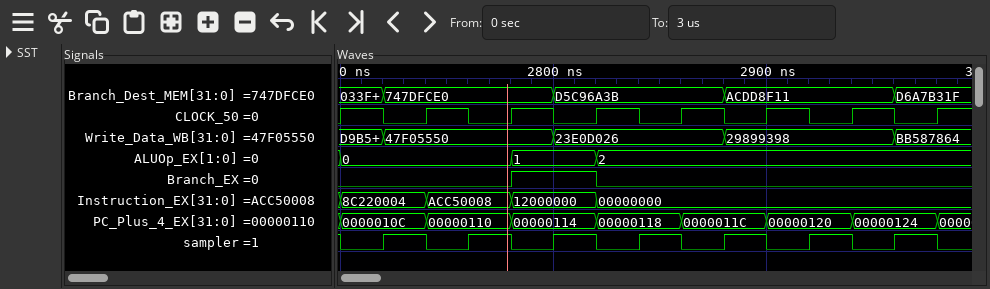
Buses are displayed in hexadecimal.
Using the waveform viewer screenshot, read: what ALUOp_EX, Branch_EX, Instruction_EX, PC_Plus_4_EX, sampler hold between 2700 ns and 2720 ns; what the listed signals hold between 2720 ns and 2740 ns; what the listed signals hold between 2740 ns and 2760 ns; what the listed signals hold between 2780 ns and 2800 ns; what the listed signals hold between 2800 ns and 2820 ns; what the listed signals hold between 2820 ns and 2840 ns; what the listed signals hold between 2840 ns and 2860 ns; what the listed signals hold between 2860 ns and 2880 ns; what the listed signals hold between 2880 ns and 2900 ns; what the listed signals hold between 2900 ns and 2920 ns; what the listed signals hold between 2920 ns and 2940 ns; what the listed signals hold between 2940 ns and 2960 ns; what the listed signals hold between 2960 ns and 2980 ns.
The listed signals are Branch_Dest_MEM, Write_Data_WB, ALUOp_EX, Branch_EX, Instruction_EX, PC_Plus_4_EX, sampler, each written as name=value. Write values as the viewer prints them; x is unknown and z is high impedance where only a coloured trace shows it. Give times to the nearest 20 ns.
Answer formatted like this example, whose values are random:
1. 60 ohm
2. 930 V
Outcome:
1. ALUOp_EX=0, Branch_EX=0, Instruction_EX=8C220004, PC_Plus_4_EX=0000010C, sampler=0
2. Branch_Dest_MEM=747DFCE0, Write_Data_WB=47F05550, ALUOp_EX=0, Branch_EX=0, Instruction_EX=8C220004, PC_Plus_4_EX=0000010C, sampler=1
3. Branch_Dest_MEM=747DFCE0, Write_Data_WB=47F05550, ALUOp_EX=0, Branch_EX=0, Instruction_EX=ACC50008, PC_Plus_4_EX=00000110, sampler=0
4. Branch_Dest_MEM=747DFCE0, Write_Data_WB=47F05550, ALUOp_EX=1, Branch_EX=1, Instruction_EX=12000000, PC_Plus_4_EX=00000114, sampler=0
5. Branch_Dest_MEM=D5C96A3B, Write_Data_WB=23E0D026, ALUOp_EX=1, Branch_EX=1, Instruction_EX=12000000, PC_Plus_4_EX=00000114, sampler=1
6. Branch_Dest_MEM=D5C96A3B, Write_Data_WB=23E0D026, ALUOp_EX=2, Branch_EX=0, Instruction_EX=00000000, PC_Plus_4_EX=00000118, sampler=0
7. Branch_Dest_MEM=D5C96A3B, Write_Data_WB=23E0D026, ALUOp_EX=2, Branch_EX=0, Instruction_EX=00000000, PC_Plus_4_EX=00000118, sampler=1
8. Branch_Dest_MEM=D5C96A3B, Write_Data_WB=23E0D026, ALUOp_EX=2, Branch_EX=0, Instruction_EX=00000000, PC_Plus_4_EX=0000011C, sampler=0
9. Branch_Dest_MEM=ACDD8F11, Write_Data_WB=29899398, ALUOp_EX=2, Branch_EX=0, Instruction_EX=00000000, PC_Plus_4_EX=0000011C, sampler=1
10. Branch_Dest_MEM=ACDD8F11, Write_Data_WB=29899398, ALUOp_EX=2, Branch_EX=0, Instruction_EX=00000000, PC_Plus_4_EX=00000120, sampler=0
11. Branch_Dest_MEM=ACDD8F11, Write_Data_WB=29899398, ALUOp_EX=2, Branch_EX=0, Instruction_EX=00000000, PC_Plus_4_EX=00000120, sampler=1
12. Branch_Dest_MEM=ACDD8F11, Write_Data_WB=29899398, ALUOp_EX=2, Branch_EX=0, Instruction_EX=00000000, PC_Plus_4_EX=00000124, sampler=0
13. Branch_Dest_MEM=D6A7B31F, Write_Data_WB=BB587864, ALUOp_EX=2, Branch_EX=0, Instruction_EX=00000000, PC_Plus_4_EX=00000124, sampler=1
